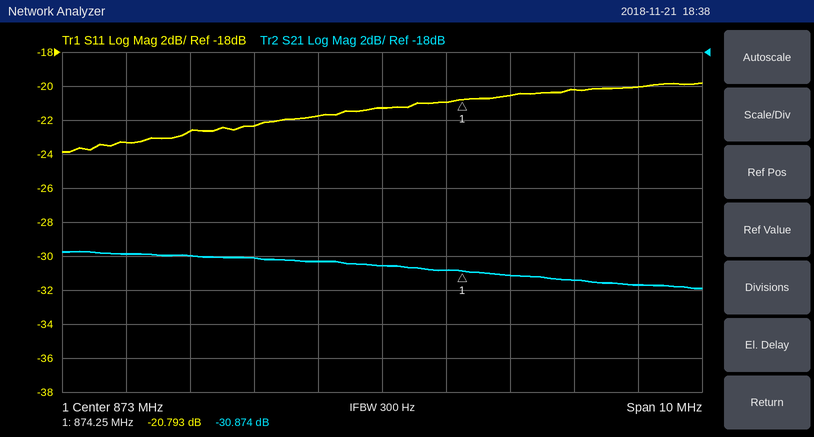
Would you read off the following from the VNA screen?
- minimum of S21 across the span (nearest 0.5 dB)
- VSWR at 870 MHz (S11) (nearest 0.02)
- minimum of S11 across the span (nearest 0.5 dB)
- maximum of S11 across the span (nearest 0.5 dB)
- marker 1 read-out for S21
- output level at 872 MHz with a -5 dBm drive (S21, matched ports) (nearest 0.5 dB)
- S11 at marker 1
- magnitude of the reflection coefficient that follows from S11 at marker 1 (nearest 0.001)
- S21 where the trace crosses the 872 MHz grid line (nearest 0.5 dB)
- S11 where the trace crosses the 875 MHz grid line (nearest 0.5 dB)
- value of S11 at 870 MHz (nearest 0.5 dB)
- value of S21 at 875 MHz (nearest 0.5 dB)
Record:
-32.0 dB
1.16
-24.0 dB
-20.0 dB
-30.874 dB
-35.5 dBm
-20.793 dB
0.091
-30.5 dB
-20.5 dB
-22.5 dB
-31.0 dB
